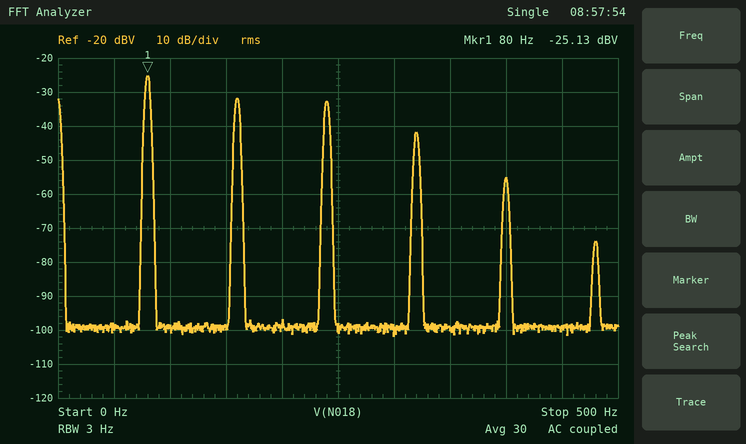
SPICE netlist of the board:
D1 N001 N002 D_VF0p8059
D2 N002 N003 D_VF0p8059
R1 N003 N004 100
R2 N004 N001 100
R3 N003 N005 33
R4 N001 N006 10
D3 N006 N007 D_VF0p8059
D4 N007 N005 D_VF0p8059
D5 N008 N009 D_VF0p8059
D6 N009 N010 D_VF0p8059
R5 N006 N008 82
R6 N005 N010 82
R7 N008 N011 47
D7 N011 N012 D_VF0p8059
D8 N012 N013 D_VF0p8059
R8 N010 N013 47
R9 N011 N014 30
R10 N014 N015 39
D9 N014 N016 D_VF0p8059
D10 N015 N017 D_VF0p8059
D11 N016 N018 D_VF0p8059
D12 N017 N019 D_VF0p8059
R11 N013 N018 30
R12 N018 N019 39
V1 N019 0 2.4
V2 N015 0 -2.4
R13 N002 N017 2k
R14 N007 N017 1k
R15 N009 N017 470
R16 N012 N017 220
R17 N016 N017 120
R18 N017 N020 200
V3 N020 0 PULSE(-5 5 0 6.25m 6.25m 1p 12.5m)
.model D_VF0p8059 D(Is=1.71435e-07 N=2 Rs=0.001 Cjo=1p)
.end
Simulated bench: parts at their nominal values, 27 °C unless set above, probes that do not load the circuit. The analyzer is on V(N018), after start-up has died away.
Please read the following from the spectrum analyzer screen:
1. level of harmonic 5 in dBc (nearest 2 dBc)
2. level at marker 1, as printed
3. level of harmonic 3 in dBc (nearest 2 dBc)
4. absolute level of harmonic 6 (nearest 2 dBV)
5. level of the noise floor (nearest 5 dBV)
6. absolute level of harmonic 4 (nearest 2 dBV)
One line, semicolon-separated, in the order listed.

-30 dBc; -25.13 dBV; -8 dBc; -74 dBV; -100 dBV; -42 dBV
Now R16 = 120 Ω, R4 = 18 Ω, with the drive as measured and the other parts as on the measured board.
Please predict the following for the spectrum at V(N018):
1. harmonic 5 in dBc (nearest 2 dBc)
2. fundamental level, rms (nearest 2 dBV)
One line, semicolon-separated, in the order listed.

-26 dBc; -24 dBV
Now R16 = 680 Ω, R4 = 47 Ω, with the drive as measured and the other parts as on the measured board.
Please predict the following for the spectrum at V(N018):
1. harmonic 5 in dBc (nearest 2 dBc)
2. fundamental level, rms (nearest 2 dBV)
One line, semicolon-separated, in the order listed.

-42 dBc; -26 dBV
